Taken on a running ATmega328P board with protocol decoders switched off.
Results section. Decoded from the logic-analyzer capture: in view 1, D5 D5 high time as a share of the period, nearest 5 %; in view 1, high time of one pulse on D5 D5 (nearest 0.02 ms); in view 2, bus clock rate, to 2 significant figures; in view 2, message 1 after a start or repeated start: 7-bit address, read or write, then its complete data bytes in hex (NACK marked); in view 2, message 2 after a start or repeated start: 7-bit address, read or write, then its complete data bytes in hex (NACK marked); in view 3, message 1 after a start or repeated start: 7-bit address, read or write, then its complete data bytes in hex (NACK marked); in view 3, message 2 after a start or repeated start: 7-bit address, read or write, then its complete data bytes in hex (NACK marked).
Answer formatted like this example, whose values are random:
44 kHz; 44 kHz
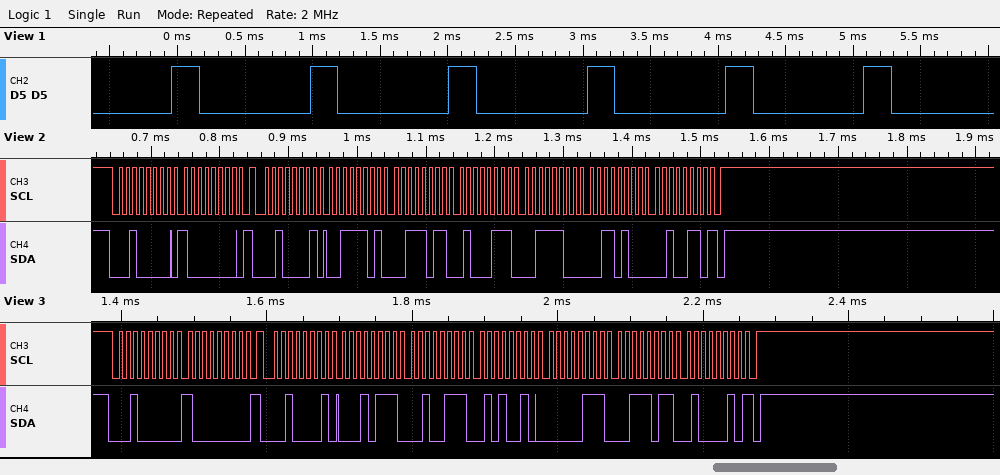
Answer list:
20 %; 0.20 ms; 100 kHz; 0x10 write: 80; 0x10 read: 3D 3B 47 3C 34 26 NACK; 0x10 write: 80; 0x10 read: 17 27 52 07 3B 42 NACK
